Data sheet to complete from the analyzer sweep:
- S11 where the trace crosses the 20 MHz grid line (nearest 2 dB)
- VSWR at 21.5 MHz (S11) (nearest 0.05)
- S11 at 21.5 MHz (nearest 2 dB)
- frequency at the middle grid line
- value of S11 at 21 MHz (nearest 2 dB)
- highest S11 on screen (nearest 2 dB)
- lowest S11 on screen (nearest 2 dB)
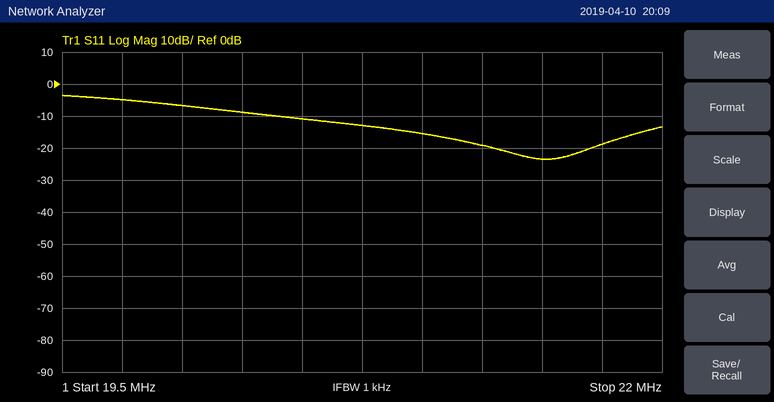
-6 dB
1.15
-24 dB
20.75 MHz
-16 dB
-4 dB
-24 dB
